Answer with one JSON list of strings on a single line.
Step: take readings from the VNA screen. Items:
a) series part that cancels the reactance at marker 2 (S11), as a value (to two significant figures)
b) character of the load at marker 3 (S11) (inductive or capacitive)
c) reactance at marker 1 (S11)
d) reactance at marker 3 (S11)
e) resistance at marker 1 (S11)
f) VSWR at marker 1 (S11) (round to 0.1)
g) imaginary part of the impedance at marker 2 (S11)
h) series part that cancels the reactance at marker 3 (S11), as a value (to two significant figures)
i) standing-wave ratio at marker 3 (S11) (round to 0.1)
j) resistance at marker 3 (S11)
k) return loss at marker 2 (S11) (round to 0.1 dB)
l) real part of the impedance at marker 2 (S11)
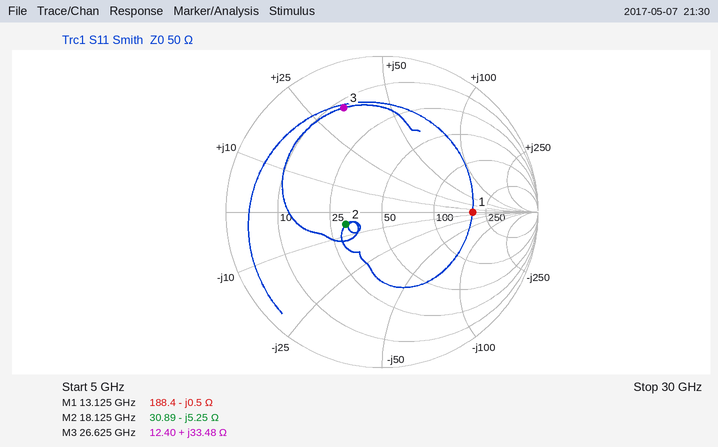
["46 pH", "inductive", "-0.5 Ω", "+33.48 Ω", "188.4 Ω", "3.8", "-5.25 Ω", "180 fF", "5.9", "12.40 Ω", "12.2 dB", "30.89 Ω"]
